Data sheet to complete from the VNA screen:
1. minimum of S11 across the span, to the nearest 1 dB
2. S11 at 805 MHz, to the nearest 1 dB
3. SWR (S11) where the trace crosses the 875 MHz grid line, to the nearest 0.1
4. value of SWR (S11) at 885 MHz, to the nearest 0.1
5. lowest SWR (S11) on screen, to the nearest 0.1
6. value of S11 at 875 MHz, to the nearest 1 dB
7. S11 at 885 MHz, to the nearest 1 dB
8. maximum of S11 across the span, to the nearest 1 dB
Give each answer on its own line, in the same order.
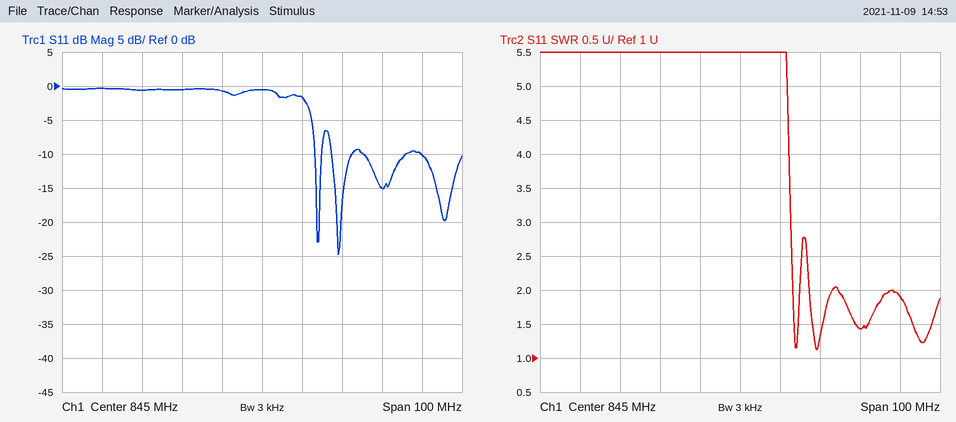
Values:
-25 dB
0 dB
1.4
1.9
1.1
-15 dB
-10 dB
0 dB
